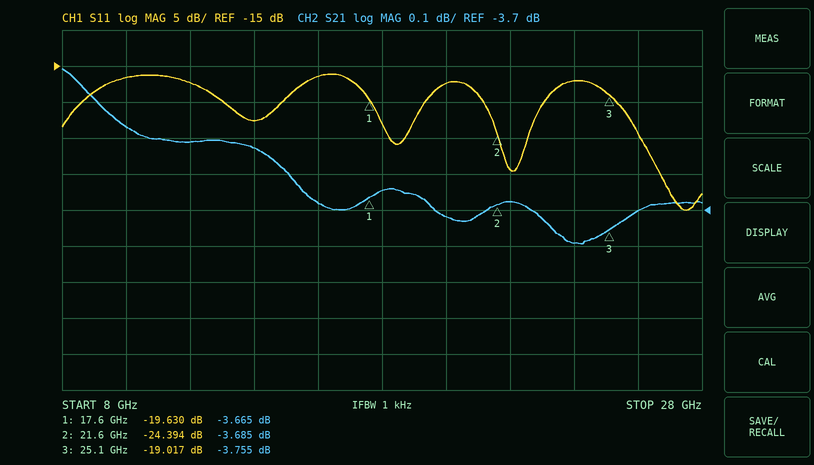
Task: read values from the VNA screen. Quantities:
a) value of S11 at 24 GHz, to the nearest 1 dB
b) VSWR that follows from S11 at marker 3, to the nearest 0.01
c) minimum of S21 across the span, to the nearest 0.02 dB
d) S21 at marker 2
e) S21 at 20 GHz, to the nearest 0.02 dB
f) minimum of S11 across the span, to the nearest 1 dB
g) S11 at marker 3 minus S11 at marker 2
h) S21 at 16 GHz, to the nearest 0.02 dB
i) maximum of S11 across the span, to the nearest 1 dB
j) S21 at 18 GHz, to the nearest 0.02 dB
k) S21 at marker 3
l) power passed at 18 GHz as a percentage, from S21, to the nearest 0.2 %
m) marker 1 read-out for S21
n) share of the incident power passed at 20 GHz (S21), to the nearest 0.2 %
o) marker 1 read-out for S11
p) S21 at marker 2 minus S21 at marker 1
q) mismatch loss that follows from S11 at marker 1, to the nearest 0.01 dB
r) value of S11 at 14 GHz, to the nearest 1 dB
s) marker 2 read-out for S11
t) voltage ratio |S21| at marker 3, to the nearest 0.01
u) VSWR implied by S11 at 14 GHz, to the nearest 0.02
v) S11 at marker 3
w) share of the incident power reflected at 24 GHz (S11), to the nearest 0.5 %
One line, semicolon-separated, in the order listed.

-17 dB; 1.25; -3.80 dB; -3.685 dB; -3.72 dB; -35 dB; 5.377 dB; -3.68 dB; -16 dB; -3.64 dB; -3.755 dB; 43.2 %; -3.665 dB; 42.4 %; -19.630 dB; -0.020 dB; 0.05 dB; -23 dB; -24.394 dB; 0.65; 1.16; -19.017 dB; 2.0 %
